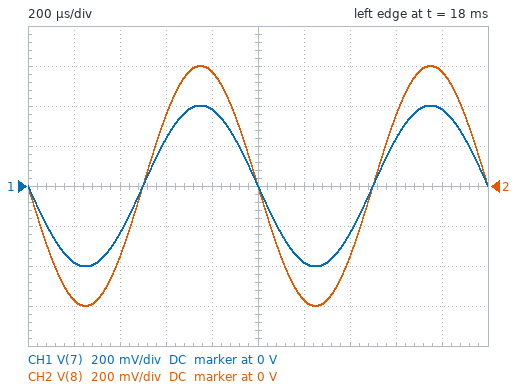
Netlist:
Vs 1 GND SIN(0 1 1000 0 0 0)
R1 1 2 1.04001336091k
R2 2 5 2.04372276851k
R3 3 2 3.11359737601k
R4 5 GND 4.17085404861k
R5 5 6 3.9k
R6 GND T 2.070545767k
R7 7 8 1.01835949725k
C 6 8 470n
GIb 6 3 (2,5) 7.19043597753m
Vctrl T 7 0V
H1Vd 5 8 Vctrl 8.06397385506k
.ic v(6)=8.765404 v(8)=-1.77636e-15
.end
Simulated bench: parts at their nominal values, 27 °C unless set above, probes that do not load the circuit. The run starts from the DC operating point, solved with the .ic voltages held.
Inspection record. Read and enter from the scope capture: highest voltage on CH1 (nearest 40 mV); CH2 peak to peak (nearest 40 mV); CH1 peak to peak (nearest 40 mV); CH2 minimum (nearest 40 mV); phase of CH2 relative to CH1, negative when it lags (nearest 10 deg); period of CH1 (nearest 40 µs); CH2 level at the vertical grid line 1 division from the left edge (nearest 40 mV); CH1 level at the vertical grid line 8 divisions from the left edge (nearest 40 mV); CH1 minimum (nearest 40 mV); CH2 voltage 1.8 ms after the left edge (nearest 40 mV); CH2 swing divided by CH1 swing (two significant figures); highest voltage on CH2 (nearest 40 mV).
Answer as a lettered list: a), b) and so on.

a) 400 mV
b) 1.20 V
c) 800 mV
d) -600 mV
e) 0 deg
f) 1.00 ms
g) -560 mV
h) 240 mV
i) -400 mV
j) 560 mV
k) 1.5
l) 600 mV
